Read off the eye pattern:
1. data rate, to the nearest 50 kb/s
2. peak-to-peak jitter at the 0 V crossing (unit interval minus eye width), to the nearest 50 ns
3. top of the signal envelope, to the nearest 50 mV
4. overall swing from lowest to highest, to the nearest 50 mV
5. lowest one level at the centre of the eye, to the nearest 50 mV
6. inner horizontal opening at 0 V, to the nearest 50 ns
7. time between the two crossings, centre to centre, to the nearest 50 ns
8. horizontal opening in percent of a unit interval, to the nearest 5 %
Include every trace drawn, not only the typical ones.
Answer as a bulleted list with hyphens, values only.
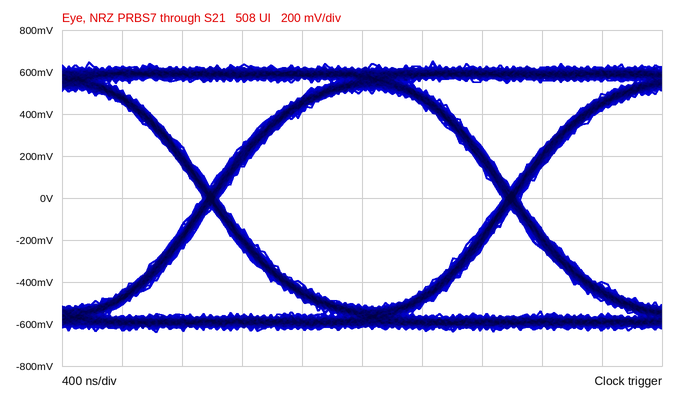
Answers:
- 500 kb/s
- 100 ns
- 650 mV
- 1.30 V
- 500 mV
- 1.90 µs
- 2.00 µs
- 95 %
